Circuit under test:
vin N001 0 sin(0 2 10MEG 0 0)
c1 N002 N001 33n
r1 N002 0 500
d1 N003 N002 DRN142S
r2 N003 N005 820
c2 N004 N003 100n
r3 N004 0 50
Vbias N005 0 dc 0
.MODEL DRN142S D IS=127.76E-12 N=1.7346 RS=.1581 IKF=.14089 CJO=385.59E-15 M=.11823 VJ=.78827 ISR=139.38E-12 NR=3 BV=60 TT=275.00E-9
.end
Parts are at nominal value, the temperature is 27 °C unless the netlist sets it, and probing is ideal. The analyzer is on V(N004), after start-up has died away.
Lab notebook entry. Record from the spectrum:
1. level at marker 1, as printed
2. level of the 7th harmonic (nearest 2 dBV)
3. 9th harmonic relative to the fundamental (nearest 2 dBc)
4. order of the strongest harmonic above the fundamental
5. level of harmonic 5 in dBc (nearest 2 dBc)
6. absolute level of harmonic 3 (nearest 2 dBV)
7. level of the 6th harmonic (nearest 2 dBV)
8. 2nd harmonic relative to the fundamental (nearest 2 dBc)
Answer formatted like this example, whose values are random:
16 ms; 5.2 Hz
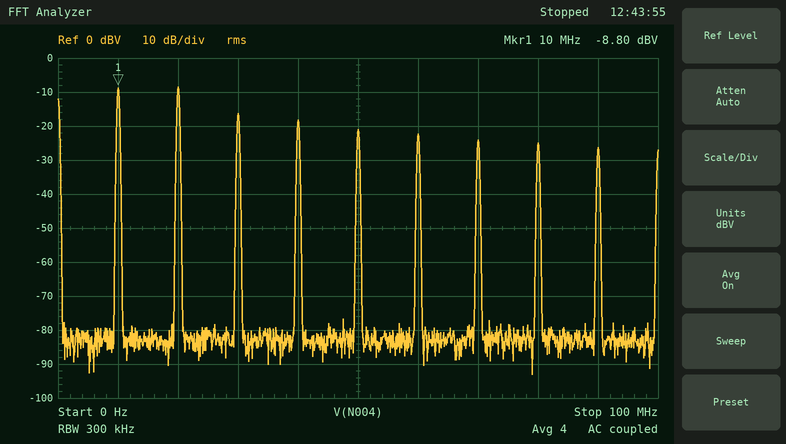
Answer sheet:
-8.80 dBV; -24 dBV; -18 dBc; 2; -12 dBc; -16 dBV; -22 dBV; 0 dBc
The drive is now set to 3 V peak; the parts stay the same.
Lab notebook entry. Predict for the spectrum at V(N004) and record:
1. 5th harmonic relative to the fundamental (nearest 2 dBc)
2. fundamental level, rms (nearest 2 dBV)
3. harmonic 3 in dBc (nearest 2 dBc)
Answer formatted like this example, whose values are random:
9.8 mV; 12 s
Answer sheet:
-14 dBc; -4 dBV; -10 dBc
